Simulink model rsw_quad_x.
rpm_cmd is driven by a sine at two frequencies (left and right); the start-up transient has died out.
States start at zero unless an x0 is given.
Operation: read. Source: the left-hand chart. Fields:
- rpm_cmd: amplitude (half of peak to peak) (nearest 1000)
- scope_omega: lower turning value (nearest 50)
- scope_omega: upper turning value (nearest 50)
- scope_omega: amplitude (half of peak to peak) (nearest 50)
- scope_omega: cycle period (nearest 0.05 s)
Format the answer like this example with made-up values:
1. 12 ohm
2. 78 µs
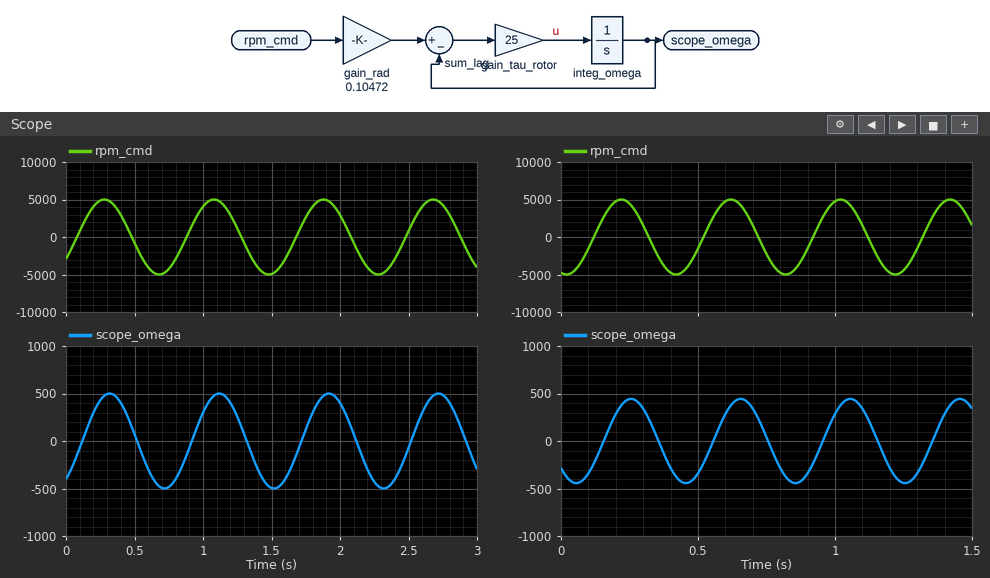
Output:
1. 5000
2. -500
3. 500
4. 500
5. 0.80 s
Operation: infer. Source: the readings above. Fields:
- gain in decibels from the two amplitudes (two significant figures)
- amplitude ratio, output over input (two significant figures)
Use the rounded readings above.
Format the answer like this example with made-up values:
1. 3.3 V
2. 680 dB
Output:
1. -20 dB
2. 0.10
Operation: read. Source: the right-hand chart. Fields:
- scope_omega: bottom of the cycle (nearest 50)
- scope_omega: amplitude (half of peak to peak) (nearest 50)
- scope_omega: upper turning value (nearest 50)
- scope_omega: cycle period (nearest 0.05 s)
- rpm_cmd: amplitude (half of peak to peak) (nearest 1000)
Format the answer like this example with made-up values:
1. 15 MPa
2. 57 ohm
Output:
1. -450
2. 450
3. 450
4. 0.40 s
5. 5000
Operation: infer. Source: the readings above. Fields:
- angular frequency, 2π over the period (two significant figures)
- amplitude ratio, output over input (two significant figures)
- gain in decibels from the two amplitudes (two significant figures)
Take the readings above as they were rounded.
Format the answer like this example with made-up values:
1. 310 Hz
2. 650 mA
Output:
1. 16 rad/s
2. 0.090
3. -21 dB
